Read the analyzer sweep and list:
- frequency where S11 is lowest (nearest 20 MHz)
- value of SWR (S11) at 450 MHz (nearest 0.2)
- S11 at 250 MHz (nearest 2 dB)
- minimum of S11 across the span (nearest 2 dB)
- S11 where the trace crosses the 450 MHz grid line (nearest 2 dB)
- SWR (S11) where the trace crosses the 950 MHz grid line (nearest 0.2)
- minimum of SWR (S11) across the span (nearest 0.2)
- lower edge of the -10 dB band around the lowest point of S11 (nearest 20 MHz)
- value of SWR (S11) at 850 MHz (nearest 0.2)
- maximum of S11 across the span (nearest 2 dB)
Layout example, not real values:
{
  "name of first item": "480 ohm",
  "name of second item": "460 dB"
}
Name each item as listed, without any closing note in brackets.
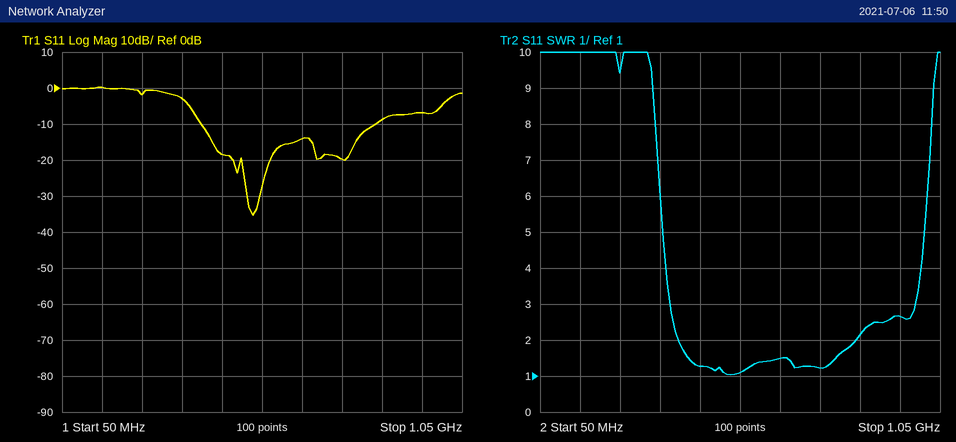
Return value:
{
  "frequency where S11 is lowest": "520 MHz",
  "value of SWR (S11) at 450 MHz": "1.2",
  "S11 at 250 MHz": "-2 dB",
  "minimum of S11 across the span": "-36 dB",
  "S11 where the trace crosses the 450 MHz grid line": "-18 dB",
  "SWR (S11) where the trace crosses the 950 MHz grid line": "2.6",
  "minimum of SWR (S11) across the span": "1.0",
  "lower edge of the -10 dB band around the lowest point of S11": "400 MHz",
  "value of SWR (S11) at 850 MHz": "2.2",
  "maximum of S11 across the span": "0 dB"
}
